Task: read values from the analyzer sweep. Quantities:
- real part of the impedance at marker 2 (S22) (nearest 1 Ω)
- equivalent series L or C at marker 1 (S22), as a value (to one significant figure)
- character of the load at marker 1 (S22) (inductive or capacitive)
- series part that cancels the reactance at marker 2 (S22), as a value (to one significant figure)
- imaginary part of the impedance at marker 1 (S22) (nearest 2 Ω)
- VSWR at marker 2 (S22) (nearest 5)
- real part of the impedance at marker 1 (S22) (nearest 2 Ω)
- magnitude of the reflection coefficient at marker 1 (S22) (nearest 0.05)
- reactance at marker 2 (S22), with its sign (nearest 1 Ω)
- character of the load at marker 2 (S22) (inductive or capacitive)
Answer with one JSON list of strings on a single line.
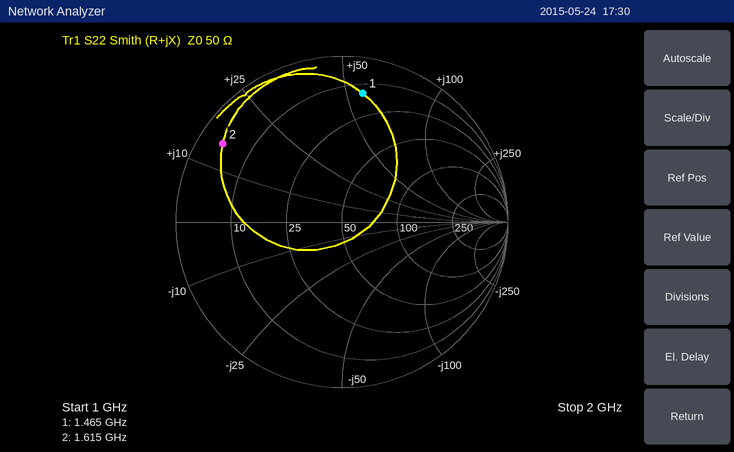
["4 Ω", "6 nH", "inductive", "7 pF", "+56 Ω", "15", "14 Ω", "0.80", "+15 Ω", "inductive"]
